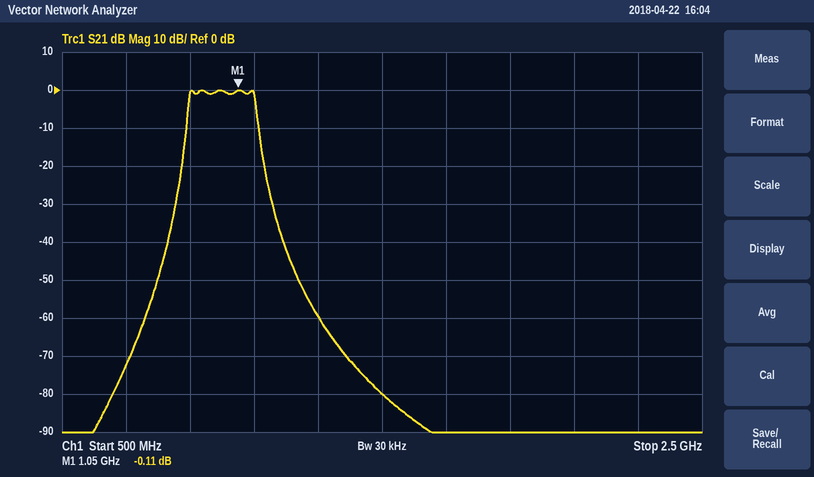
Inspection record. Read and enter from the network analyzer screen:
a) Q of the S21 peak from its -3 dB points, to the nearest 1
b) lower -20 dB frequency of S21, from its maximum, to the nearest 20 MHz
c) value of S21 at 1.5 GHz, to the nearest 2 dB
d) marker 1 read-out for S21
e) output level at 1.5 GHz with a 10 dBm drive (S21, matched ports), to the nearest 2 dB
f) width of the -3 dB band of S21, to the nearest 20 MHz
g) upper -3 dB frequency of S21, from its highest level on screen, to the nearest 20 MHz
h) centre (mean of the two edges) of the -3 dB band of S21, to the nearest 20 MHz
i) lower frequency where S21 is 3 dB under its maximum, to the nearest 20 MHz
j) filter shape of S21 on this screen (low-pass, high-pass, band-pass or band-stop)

5
880 MHz
-80 dB
-0.11 dB
-70 dBm
200 MHz
1.10 GHz
1.00 GHz
900 MHz
band-pass
